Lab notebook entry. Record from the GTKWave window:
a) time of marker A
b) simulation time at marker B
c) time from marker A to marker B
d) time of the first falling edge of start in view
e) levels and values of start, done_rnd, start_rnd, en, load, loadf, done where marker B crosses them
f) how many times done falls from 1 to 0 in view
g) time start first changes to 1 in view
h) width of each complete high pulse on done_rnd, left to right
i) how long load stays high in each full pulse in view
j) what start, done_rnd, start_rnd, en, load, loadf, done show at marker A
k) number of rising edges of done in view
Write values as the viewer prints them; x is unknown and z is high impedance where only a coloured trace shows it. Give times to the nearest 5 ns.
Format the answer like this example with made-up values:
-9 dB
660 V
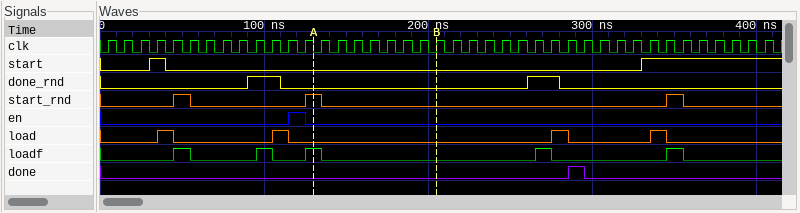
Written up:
130 ns
205 ns
75 ns
40 ns
start=0, done_rnd=0, start_rnd=0, en=0, load=0, loadf=0, done=0
1
30 ns
20 ns, 20 ns
10 ns, 10 ns, 10 ns, 10 ns
start=0, done_rnd=0, start_rnd=1, en=0, load=0, loadf=1, done=0
1
